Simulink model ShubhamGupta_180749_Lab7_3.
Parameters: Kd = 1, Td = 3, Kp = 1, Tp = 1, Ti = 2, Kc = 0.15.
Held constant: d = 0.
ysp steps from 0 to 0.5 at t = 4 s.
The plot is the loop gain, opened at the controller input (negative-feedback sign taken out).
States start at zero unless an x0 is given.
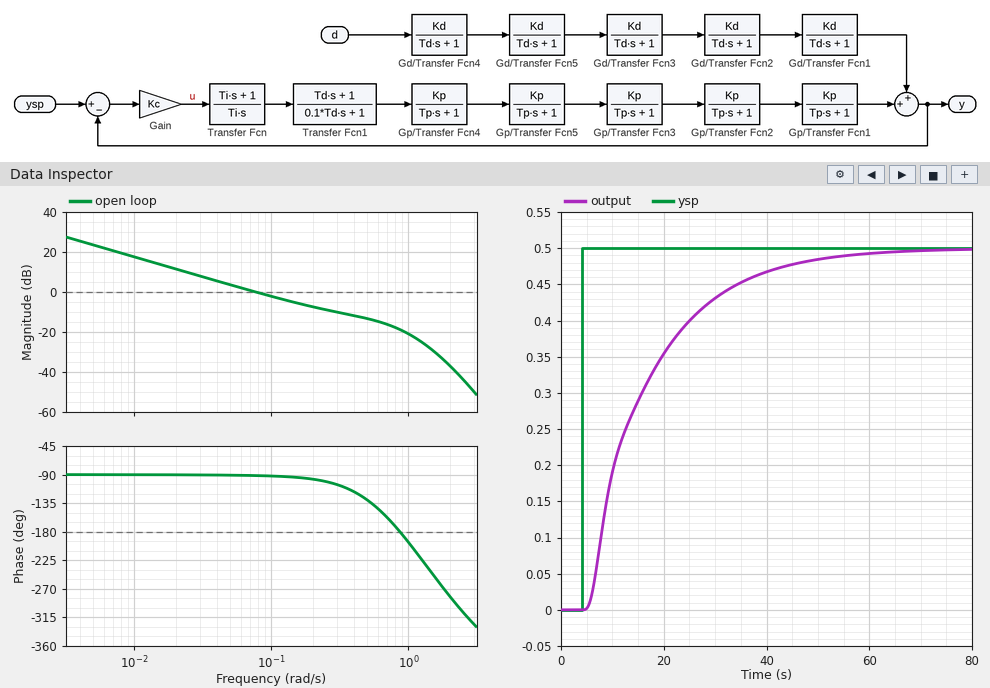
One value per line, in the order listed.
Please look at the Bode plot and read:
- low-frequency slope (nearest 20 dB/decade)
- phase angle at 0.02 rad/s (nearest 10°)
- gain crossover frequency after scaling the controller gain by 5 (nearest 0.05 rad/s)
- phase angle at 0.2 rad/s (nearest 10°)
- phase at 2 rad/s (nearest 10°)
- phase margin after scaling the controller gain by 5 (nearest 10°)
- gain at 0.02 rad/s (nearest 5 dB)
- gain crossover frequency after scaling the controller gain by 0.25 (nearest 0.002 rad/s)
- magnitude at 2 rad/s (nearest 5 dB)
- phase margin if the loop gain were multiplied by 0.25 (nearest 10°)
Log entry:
-20 dB/decade
-90°
0.55 rad/s
-100°
-280°
40°
10 dB
0.018 rad/s
-35 dB
90°
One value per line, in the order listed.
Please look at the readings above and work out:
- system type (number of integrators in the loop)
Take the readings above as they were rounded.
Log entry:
1
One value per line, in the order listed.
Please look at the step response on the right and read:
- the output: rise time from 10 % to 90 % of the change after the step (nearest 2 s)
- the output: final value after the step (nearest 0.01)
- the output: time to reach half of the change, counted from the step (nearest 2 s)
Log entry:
28 s
0.50
8 s
